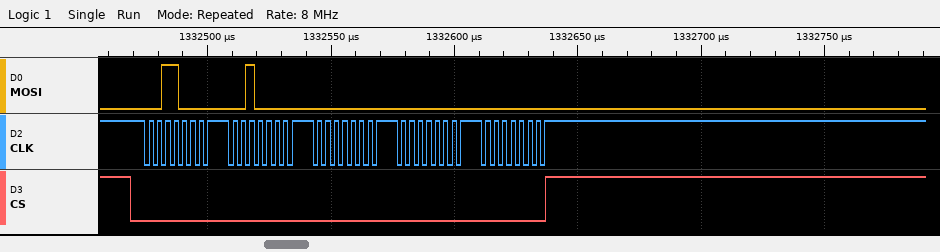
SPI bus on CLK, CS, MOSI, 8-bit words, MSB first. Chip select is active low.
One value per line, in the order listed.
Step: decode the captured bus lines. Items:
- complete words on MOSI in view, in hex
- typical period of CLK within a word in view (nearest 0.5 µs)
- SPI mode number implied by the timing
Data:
30, 20, 00, 00, 00
3.5 µs
3
